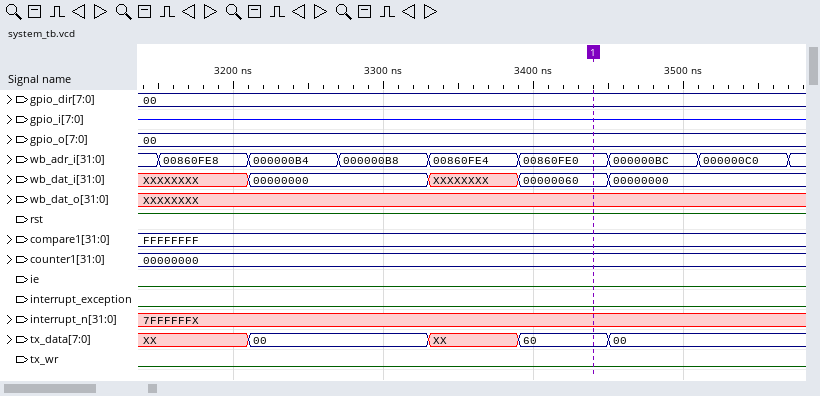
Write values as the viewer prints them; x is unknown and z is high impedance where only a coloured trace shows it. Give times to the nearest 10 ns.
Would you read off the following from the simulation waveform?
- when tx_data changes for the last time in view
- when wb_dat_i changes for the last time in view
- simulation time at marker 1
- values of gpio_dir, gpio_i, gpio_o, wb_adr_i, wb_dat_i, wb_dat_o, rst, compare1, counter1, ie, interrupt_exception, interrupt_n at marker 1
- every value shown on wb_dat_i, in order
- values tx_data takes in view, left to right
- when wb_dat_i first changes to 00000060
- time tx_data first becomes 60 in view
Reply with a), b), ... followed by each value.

a) 3450 ns
b) 3450 ns
c) 3440 ns
d) gpio_dir=00, gpio_i=z, gpio_o=00, wb_adr_i=00860FE0, wb_dat_i=00000060, wb_dat_o=XXXXXXXX, rst=1, compare1=FFFFFFFF, counter1=00000000, ie=0, interrupt_exception=0, interrupt_n=7FFFFFFX
e) XXXXXXXX, 00000000, XXXXXXXX, 00000060, 00000000
f) XX, 00, XX, 60, 00
g) 3390 ns
h) 3390 ns
